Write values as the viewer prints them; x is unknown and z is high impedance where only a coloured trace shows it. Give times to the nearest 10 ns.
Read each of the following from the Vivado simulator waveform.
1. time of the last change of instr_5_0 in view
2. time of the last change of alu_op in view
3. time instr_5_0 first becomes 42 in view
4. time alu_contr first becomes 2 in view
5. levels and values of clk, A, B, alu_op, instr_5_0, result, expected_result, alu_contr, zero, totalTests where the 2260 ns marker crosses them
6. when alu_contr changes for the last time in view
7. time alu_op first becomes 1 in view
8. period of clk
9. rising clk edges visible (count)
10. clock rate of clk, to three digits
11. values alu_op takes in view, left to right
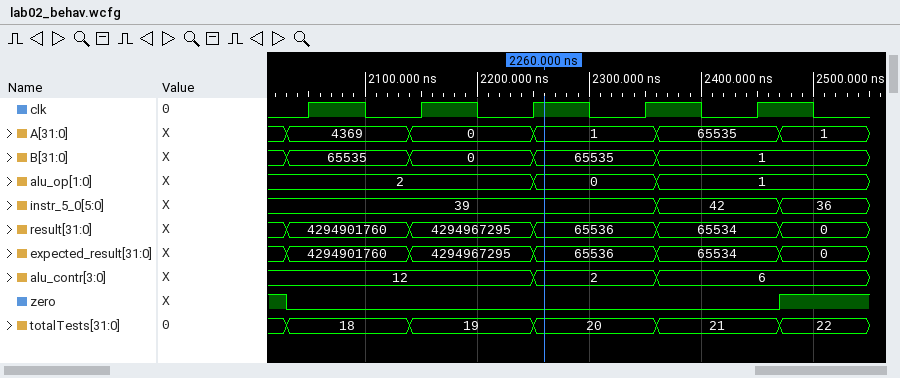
2470 ns
2360 ns
2360 ns
2250 ns
clk=1, A=1, B=65535, alu_op=0, instr_5_0=39, result=65536, expected_result=65536, alu_contr=2, zero=0, totalTests=20
2360 ns
2360 ns
100 ns
5
10.0 MHz
2, 0, 1
